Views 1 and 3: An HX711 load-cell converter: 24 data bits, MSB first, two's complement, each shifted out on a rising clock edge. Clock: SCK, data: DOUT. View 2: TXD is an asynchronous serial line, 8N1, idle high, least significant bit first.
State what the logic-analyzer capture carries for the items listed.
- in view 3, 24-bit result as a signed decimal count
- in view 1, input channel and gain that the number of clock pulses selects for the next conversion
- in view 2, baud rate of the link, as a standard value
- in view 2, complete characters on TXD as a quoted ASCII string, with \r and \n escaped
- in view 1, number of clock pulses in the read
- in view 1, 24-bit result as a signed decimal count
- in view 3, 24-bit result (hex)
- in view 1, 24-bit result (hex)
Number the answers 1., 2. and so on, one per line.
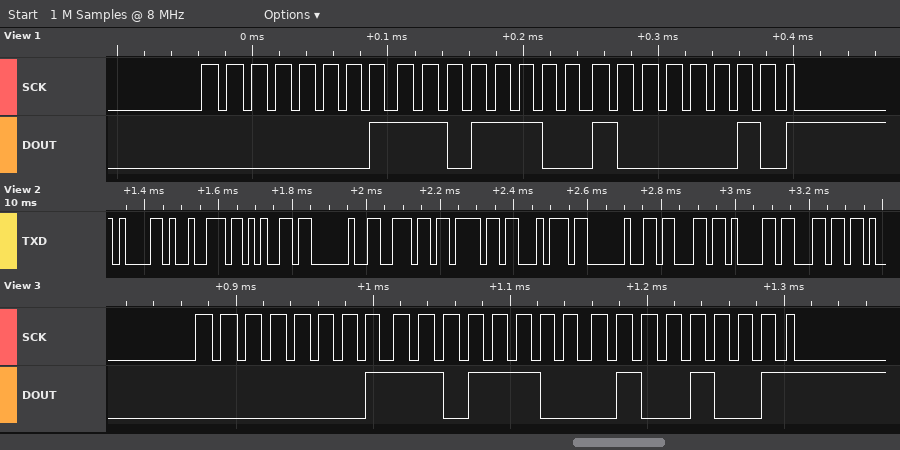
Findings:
1. 121929
2. channel A, gain 128
3. 57600 baud
4. "are not cal"
5. 25
6. 121986
7. 0x01DC49
8. 0x01DC82
